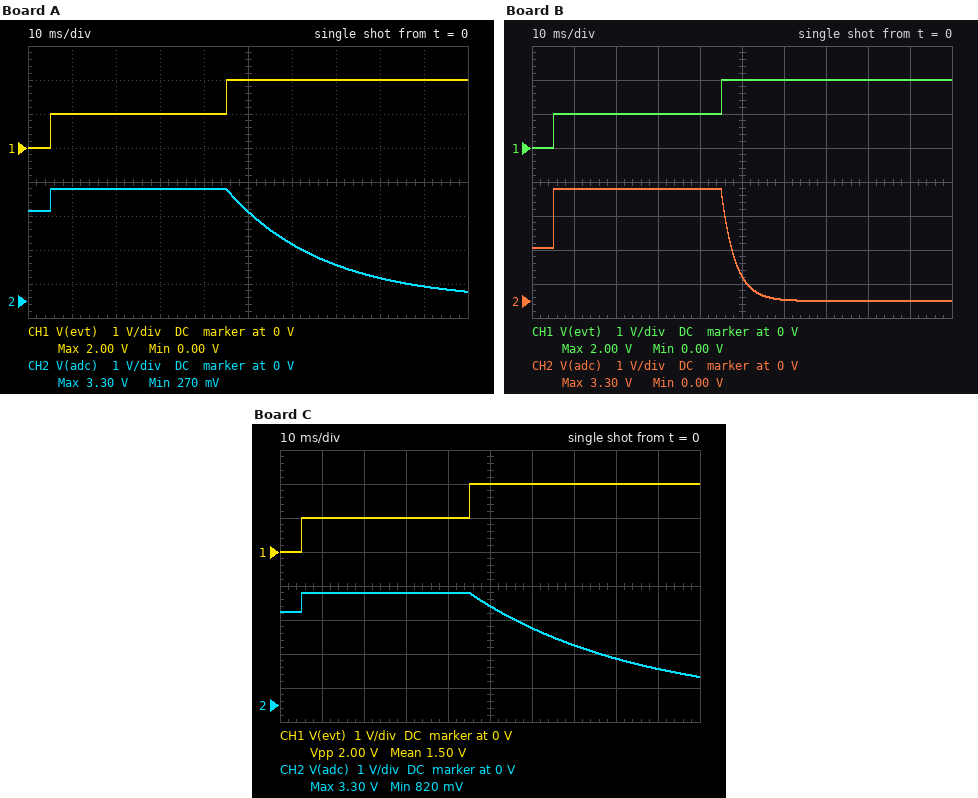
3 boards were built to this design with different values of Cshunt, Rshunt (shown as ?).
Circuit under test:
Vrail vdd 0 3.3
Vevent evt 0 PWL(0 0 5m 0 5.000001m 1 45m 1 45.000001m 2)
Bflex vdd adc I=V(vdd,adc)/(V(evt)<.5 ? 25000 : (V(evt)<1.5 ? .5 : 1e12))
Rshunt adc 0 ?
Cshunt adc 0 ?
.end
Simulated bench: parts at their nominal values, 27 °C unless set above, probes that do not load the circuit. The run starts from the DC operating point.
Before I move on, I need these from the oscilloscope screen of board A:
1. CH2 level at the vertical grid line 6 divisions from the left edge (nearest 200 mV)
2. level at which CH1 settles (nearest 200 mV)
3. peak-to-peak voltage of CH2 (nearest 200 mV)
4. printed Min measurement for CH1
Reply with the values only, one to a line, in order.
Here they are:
1.6 V
2.0 V
3.0 V
0.00 V
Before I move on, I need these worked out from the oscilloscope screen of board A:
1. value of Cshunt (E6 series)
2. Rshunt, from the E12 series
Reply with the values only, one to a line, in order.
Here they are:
220 nF
100 kΩ
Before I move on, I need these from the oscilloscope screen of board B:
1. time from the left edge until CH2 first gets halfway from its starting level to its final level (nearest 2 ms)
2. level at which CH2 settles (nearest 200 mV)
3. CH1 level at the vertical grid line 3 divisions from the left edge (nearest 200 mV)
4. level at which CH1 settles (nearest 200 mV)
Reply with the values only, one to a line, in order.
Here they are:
50 ms
0 V
1.0 V
2.0 V
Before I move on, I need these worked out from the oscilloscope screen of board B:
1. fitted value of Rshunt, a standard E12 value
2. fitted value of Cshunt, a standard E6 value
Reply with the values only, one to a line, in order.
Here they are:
22 kΩ
150 nF
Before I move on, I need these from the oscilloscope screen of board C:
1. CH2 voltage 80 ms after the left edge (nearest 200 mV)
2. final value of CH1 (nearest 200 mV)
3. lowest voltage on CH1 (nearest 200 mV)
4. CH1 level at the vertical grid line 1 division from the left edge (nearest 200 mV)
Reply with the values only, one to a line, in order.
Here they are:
1.4 V
2.0 V
0 V
1.0 V
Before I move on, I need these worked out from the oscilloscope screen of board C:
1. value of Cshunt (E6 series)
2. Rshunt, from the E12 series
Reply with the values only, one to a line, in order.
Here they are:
330 nF
120 kΩ
